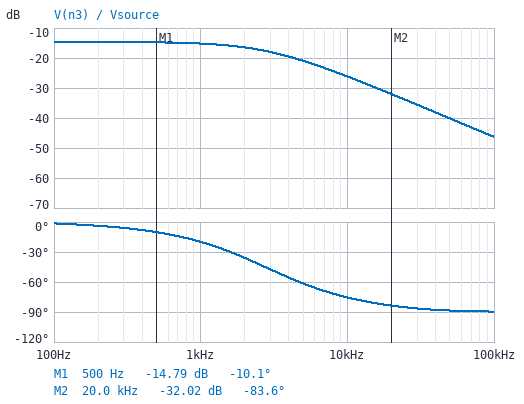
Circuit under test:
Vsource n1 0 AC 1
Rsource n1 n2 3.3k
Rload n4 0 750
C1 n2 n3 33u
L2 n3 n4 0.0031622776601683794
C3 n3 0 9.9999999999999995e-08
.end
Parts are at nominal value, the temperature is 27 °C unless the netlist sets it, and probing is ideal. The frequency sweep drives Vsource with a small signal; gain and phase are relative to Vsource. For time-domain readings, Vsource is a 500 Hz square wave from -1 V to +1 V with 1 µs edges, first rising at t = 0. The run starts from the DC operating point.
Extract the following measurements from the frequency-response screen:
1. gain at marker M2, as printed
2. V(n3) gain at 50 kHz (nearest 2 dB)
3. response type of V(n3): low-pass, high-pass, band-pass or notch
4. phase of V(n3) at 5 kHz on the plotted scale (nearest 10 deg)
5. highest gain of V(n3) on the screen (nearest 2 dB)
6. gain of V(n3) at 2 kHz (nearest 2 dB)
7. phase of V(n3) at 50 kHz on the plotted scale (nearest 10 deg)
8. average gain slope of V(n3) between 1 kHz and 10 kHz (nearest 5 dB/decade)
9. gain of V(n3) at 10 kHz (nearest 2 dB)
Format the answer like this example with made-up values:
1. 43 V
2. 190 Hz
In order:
1. -32.02 dB
2. -40 dB
3. low-pass
4. -60 deg
5. -14 dB
6. -16 dB
7. -90 deg
8. -10 dB/decade
9. -26 dB
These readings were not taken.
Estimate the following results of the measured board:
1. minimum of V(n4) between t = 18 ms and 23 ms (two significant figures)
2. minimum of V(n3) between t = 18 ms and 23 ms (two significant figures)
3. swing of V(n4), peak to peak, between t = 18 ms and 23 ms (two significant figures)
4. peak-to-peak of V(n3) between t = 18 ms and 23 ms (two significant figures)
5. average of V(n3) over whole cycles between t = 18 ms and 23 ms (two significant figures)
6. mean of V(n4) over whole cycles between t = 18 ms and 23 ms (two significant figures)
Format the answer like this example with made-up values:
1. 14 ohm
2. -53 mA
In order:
1. -28 mV
2. -28 mV
3. 370 mV
4. 370 mV
5. 160 mV
6. 160 mV
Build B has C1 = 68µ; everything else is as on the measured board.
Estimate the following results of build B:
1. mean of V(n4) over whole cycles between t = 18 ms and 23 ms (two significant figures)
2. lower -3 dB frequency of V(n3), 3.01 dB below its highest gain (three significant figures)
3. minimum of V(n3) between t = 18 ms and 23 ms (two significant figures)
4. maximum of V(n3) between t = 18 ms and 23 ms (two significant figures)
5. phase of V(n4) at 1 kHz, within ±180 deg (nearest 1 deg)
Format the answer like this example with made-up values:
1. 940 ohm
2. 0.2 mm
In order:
1. 170 mV
2. 578 mHz
3. -14 mV
4. 360 mV
5. -21 deg
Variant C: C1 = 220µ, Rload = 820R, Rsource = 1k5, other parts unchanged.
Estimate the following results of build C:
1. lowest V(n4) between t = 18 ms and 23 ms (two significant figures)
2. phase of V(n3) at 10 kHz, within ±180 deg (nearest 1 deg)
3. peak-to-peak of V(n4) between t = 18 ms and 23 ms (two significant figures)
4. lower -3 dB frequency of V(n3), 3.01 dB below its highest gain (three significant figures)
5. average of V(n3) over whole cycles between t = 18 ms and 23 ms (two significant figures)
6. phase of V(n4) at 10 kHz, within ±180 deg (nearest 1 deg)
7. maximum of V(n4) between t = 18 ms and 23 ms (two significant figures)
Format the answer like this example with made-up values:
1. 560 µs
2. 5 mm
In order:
1. -15 mV
2. -73 deg
3. 710 mV
4. 312 mHz
5. 340 mV
6. -87 deg
7. 690 mV
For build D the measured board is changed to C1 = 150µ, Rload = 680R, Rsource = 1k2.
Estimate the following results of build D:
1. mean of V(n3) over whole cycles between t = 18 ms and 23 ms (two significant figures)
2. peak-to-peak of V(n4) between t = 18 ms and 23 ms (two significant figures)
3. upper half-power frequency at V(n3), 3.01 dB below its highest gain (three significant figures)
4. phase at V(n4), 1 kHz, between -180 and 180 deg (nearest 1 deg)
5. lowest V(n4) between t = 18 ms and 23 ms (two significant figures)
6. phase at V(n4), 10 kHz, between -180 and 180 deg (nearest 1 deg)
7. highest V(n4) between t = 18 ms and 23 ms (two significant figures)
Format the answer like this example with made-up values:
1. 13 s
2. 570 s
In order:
1. 340 mV
2. 730 mV
3. 3.97 kHz
4. -16 deg
5. -27 mV
6. -86 deg
7. 700 mV
